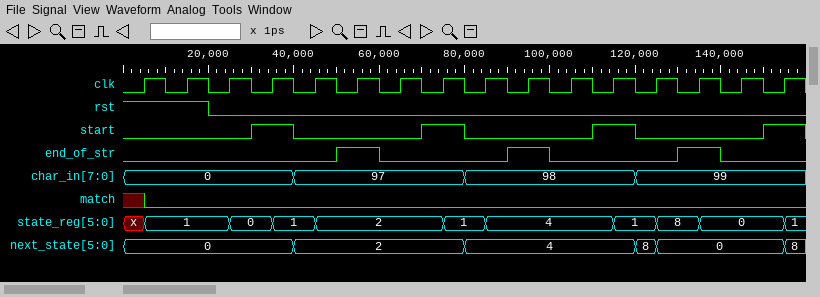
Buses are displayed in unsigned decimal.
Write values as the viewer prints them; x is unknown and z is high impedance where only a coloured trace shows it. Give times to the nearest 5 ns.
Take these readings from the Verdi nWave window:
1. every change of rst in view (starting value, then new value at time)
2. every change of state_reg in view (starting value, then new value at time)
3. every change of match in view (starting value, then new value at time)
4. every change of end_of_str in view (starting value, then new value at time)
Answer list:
1, 0 at 20 ns
x, 1 at 5 ns, 0 at 25 ns, 1 at 35 ns, 2 at 45 ns, 1 at 75 ns, 4 at 85 ns, 1 at 115 ns, 8 at 125 ns, 0 at 135 ns, 1 at 155 ns
x, 0 at 5 ns
0, 1 at 50 ns, 0 at 60 ns, 1 at 90 ns, 0 at 100 ns, 1 at 130 ns, 0 at 140 ns
